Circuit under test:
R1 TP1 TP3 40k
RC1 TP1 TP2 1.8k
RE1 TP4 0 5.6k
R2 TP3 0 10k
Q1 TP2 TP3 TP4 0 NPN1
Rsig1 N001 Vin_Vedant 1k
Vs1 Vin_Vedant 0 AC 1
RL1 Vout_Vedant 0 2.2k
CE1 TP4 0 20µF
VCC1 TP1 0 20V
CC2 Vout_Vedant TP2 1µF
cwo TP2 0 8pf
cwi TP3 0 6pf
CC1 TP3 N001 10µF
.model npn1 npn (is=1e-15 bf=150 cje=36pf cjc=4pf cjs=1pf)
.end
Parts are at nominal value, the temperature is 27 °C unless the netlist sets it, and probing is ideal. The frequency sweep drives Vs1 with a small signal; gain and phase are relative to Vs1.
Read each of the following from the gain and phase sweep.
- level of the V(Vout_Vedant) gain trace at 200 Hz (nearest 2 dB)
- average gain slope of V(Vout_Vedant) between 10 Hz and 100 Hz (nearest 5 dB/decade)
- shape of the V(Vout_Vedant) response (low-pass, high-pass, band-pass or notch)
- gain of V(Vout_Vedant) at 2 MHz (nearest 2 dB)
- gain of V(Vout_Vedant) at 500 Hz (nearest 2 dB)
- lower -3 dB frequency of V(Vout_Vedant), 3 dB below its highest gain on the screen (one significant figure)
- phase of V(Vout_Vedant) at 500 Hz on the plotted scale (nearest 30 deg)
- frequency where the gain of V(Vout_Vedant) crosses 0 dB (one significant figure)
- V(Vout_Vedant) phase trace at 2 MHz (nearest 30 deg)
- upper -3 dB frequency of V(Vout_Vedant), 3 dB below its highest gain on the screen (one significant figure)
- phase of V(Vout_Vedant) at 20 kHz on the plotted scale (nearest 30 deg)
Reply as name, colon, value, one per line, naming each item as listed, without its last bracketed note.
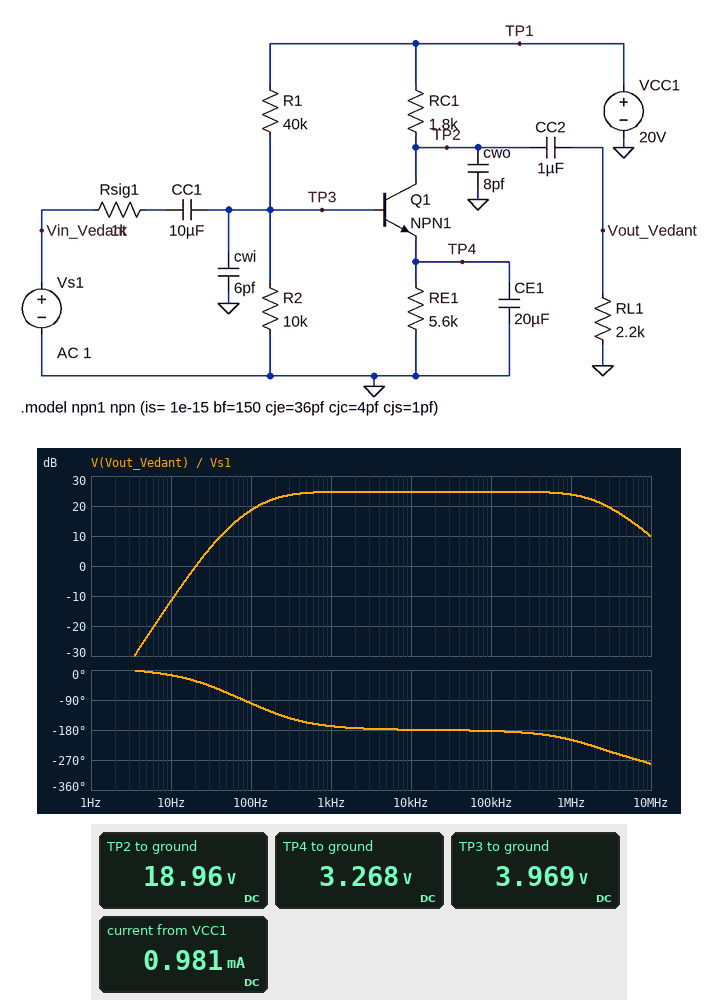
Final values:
level of the V(Vout_Vedant) gain trace at 200 Hz: 22 dB
average gain slope of V(Vout_Vedant) between 10 Hz and 100 Hz: 30 dB/decade
shape of the V(Vout_Vedant) response: band-pass
gain of V(Vout_Vedant) at 2 MHz: 22 dB
gain of V(Vout_Vedant) at 500 Hz: 24 dB
lower -3 dB frequency of V(Vout_Vedant), 3 dB below its highest gain on the screen: 200 Hz
phase of V(Vout_Vedant) at 500 Hz on the plotted scale: -150 deg
frequency where the gain of V(Vout_Vedant) crosses 0 dB: 20 Hz
V(Vout_Vedant) phase trace at 2 MHz: -240 deg
upper -3 dB frequency of V(Vout_Vedant), 3 dB below its highest gain on the screen: 2 MHz
phase of V(Vout_Vedant) at 20 kHz on the plotted scale: -180 deg
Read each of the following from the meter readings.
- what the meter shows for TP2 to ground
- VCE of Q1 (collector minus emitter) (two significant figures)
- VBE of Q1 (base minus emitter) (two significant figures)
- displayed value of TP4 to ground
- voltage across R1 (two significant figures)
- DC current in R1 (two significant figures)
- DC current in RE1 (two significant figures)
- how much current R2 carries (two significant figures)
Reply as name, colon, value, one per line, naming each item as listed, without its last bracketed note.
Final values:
what the meter shows for TP2 to ground: 18.96 V
VCE of Q1 (collector minus emitter): 16 V
VBE of Q1 (base minus emitter): 700 mV
displayed value of TP4 to ground: 3.268 V
voltage across R1: 16 V
DC current in R1: 400 µA
DC current in RE1: 580 µA
how much current R2 carries: 400 µA
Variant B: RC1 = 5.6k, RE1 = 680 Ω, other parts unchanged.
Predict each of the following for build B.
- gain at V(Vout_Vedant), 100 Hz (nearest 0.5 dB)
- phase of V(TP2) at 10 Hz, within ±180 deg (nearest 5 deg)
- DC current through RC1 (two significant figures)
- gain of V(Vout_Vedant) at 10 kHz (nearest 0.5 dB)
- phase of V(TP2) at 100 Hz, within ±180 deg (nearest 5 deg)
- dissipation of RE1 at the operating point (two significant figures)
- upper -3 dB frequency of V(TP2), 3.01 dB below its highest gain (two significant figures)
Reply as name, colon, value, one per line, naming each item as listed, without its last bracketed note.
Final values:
gain at V(Vout_Vedant), 100 Hz: -15.5 dB
phase of V(TP2) at 10 Hz, within ±180 deg: -5 deg
DC current through RC1: 3.2 mA
gain of V(Vout_Vedant) at 10 kHz: -13.0 dB
phase of V(TP2) at 100 Hz, within ±180 deg: -145 deg
dissipation of RE1 at the operating point: 7.3 mW
upper -3 dB frequency of V(TP2), 3.01 dB below its highest gain: 78 MHz
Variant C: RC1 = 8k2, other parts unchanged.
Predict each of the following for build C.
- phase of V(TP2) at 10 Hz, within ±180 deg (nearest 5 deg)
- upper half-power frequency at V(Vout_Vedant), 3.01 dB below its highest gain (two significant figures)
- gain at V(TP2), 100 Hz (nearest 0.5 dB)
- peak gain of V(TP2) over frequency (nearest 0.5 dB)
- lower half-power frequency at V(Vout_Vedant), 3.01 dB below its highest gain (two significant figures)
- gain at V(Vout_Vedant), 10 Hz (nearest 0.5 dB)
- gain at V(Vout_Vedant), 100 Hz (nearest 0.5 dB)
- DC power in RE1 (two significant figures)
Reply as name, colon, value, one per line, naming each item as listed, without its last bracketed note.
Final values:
phase of V(TP2) at 10 Hz, within ±180 deg: -115 deg
upper half-power frequency at V(Vout_Vedant), 3.01 dB below its highest gain: 1.4 MHz
gain at V(TP2), 100 Hz: 26.0 dB
peak gain of V(TP2) over frequency: 29.5 dB
lower half-power frequency at V(Vout_Vedant), 3.01 dB below its highest gain: 160 Hz
gain at V(Vout_Vedant), 10 Hz: 0 dB
gain at V(Vout_Vedant), 100 Hz: 24.0 dB
DC power in RE1: 1.9 mW
